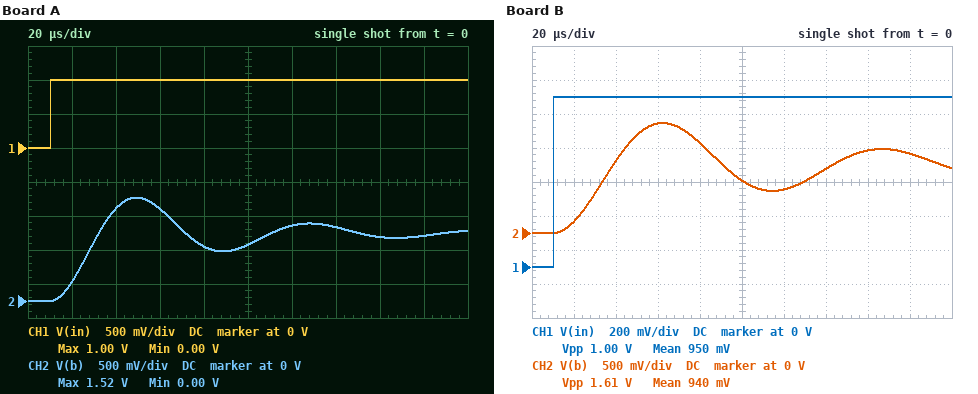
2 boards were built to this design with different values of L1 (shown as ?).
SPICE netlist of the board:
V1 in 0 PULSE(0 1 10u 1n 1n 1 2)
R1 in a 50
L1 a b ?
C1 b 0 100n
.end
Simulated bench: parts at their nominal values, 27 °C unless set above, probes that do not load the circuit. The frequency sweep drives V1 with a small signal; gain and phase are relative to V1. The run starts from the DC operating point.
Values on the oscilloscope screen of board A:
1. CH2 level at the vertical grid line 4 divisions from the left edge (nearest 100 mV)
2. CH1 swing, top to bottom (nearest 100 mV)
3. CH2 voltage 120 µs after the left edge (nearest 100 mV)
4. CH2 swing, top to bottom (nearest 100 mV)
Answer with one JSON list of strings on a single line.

["800 mV", "1.0 V", "1.1 V", "1.5 V"]
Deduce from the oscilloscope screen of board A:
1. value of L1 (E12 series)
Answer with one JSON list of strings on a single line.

["1.5 mH"]
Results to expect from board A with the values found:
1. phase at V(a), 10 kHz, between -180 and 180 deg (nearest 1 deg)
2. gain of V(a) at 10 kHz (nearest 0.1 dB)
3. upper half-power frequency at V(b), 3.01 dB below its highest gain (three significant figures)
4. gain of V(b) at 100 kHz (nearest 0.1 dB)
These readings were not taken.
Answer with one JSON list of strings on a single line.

["-38 deg", "-2.0 dB", "14.9 kHz", "-35.3 dB"]
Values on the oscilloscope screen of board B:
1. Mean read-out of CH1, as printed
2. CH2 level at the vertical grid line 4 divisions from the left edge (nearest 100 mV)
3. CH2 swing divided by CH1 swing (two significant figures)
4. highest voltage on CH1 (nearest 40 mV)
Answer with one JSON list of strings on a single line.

["950 mV", "1.3 V", "1.6", "1.00 V"]
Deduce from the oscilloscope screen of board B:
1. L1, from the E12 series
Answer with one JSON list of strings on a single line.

["2.7 mH"]
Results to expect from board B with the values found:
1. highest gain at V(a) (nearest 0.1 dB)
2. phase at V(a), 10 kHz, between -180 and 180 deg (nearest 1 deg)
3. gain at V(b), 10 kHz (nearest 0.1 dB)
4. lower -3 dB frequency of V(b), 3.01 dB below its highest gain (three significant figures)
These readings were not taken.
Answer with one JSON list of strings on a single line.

["0 dB", "78 deg", "9.9 dB", "7.83 kHz"]
